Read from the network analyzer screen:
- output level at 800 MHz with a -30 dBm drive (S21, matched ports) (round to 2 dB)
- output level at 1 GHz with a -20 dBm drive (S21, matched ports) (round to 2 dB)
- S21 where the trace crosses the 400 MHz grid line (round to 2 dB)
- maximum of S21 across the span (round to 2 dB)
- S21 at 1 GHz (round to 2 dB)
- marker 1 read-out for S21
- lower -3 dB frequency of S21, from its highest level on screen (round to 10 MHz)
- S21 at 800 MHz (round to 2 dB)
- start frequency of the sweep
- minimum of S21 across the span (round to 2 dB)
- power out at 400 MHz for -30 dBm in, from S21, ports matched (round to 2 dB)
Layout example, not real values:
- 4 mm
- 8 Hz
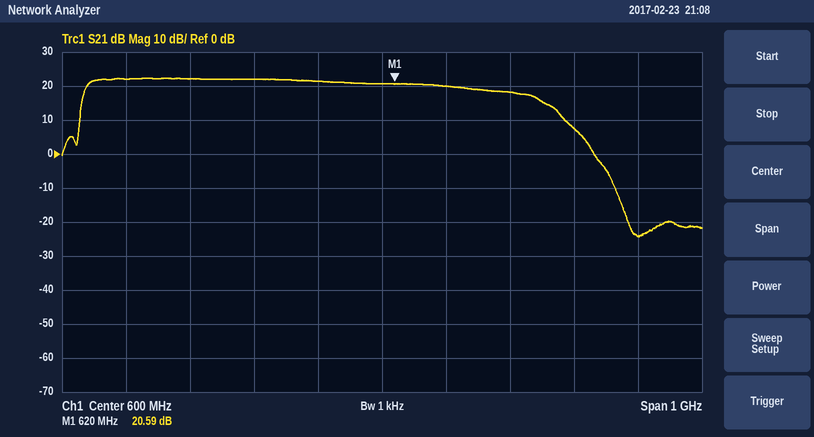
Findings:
- -12 dBm
- -44 dBm
- 22 dB
- 22 dB
- -24 dB
- 20.59 dB
- 140 MHz
- 18 dB
- 100 MHz
- -24 dB
- -8 dBm
